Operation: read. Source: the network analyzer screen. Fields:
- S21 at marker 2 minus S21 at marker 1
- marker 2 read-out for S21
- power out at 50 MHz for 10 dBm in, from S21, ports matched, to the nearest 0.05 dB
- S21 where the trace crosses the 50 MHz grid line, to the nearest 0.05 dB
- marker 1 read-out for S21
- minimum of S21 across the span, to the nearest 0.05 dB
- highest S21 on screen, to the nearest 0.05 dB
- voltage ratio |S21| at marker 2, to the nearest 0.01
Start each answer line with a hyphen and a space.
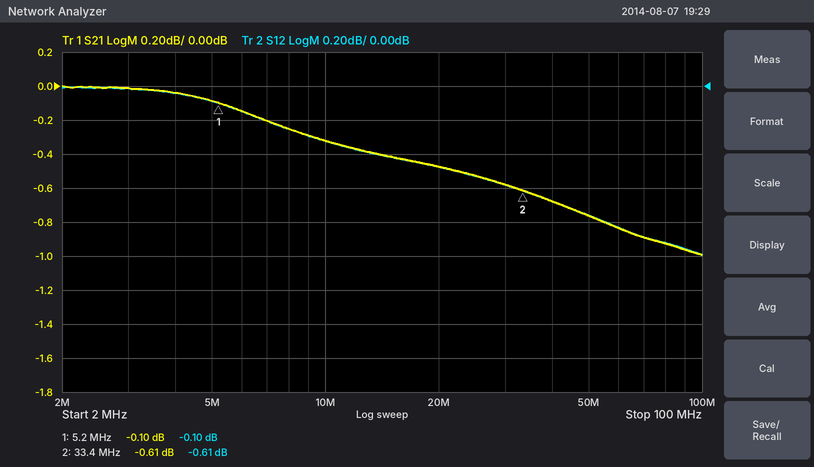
- -0.51 dB
- -0.61 dB
- 9.25 dBm
- -0.75 dB
- -0.10 dB
- -1.00 dB
- 0.00 dB
- 0.93
